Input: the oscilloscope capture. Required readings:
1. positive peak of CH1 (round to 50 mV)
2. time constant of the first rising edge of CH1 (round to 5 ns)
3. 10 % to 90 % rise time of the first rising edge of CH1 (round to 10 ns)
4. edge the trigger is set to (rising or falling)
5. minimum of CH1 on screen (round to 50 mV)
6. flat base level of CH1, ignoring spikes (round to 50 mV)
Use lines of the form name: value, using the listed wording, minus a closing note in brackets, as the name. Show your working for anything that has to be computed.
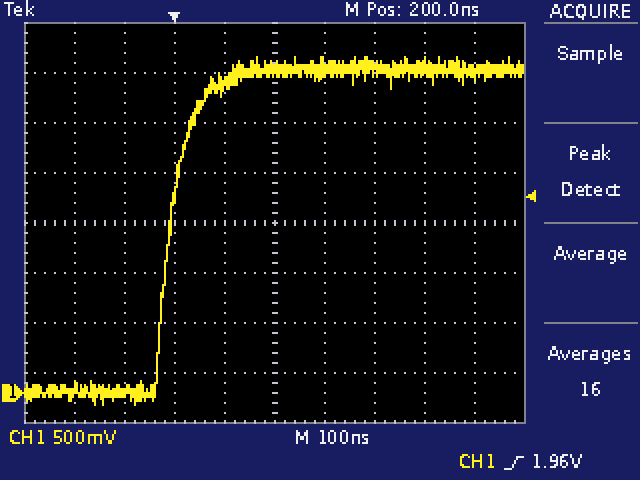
positive peak of CH1: 3.35 V
time constant of the first rising edge of CH1: 90 ns / 2.2 ≈ 40.9 ns, so 40 ns to the nearest 5 ns
10 % to 90 % rise time of the first rising edge of CH1: 90 ns
edge the trigger is set to: rising
minimum of CH1 on screen: -100 mV
flat base level of CH1, ignoring spikes: 0 mV
